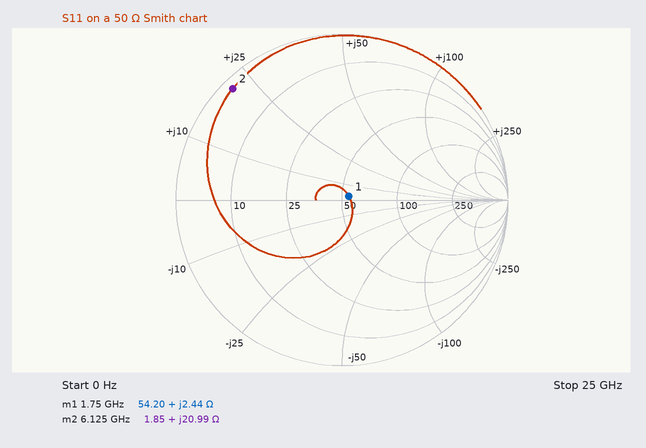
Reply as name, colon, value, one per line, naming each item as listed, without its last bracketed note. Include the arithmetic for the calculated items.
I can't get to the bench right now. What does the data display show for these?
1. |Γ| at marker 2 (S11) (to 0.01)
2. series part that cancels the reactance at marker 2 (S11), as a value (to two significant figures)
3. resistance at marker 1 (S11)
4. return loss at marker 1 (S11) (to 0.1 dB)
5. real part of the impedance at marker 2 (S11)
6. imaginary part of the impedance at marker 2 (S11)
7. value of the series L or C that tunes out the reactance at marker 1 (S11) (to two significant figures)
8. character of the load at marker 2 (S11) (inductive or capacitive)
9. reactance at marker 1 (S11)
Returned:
|Γ| at marker 2 (S11): 0.94
series part that cancels the reactance at marker 2 (S11), as a value: C = 1/(2π × 6.125 GHz × 20.99 Ω) ≈ 1.2 pF
resistance at marker 1: 54.20 Ω
return loss at marker 1 (S11): 26.6 dB
real part of the impedance at marker 2: 1.85 Ω
imaginary part of the impedance at marker 2: +20.99 Ω
value of the series L or C that tunes out the reactance at marker 1 (S11): C = 1/(2π × 1.75 GHz × 2.44 Ω) ≈ 37 pF
character of the load at marker 2 (S11): inductive
reactance at marker 1: +2.44 Ω
